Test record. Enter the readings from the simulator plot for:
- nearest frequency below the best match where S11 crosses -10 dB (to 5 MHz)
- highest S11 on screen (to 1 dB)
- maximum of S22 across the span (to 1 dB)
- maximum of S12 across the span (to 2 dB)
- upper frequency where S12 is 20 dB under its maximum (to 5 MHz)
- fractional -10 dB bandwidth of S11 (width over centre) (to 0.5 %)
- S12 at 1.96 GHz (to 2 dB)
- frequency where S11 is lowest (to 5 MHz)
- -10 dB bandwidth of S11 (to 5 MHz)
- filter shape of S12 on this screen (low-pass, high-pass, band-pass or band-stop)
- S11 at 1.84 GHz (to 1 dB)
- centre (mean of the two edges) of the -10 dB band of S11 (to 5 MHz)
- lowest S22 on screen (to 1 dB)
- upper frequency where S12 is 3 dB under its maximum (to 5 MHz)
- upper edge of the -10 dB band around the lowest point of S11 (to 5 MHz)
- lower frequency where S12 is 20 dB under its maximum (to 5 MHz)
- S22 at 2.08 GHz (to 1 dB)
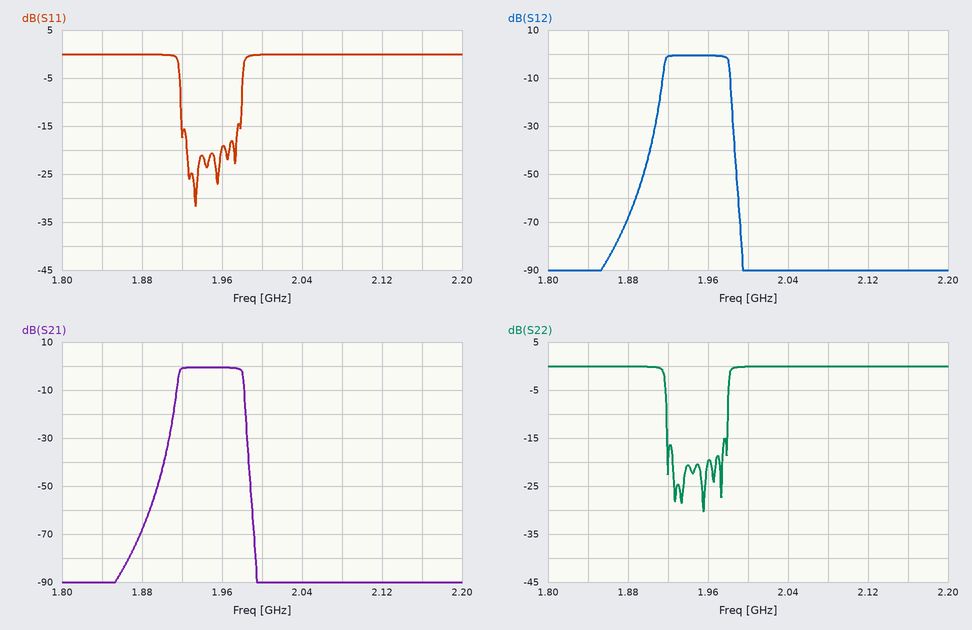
1.920 GHz
0 dB
0 dB
0 dB
1.985 GHz
3.0 %
0 dB
1.935 GHz
60 MHz
band-pass
0 dB
1.950 GHz
-30 dB
1.980 GHz
1.980 GHz
1.910 GHz
0 dB
